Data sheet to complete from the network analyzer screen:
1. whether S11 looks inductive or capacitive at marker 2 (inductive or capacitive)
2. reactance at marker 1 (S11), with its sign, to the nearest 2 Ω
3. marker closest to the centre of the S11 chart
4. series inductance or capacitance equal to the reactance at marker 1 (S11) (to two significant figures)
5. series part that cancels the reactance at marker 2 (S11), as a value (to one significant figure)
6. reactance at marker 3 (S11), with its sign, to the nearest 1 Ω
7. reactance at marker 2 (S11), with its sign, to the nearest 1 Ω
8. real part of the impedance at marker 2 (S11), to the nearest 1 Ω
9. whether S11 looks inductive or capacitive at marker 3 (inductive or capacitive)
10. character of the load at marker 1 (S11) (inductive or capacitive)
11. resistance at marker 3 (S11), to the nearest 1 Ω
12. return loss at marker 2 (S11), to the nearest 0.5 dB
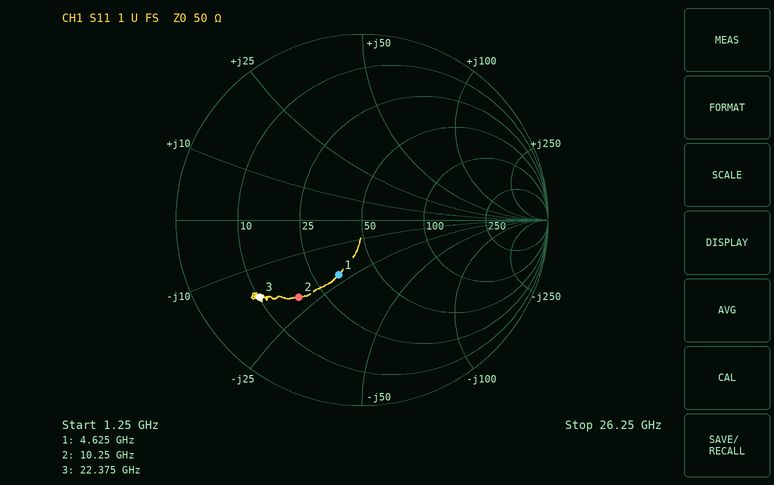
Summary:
capacitive
-22 Ω
marker 1
1.6 pF
300 pH
-16 Ω
-21 Ω
18 Ω
capacitive
capacitive
10 Ω
5.5 dB
